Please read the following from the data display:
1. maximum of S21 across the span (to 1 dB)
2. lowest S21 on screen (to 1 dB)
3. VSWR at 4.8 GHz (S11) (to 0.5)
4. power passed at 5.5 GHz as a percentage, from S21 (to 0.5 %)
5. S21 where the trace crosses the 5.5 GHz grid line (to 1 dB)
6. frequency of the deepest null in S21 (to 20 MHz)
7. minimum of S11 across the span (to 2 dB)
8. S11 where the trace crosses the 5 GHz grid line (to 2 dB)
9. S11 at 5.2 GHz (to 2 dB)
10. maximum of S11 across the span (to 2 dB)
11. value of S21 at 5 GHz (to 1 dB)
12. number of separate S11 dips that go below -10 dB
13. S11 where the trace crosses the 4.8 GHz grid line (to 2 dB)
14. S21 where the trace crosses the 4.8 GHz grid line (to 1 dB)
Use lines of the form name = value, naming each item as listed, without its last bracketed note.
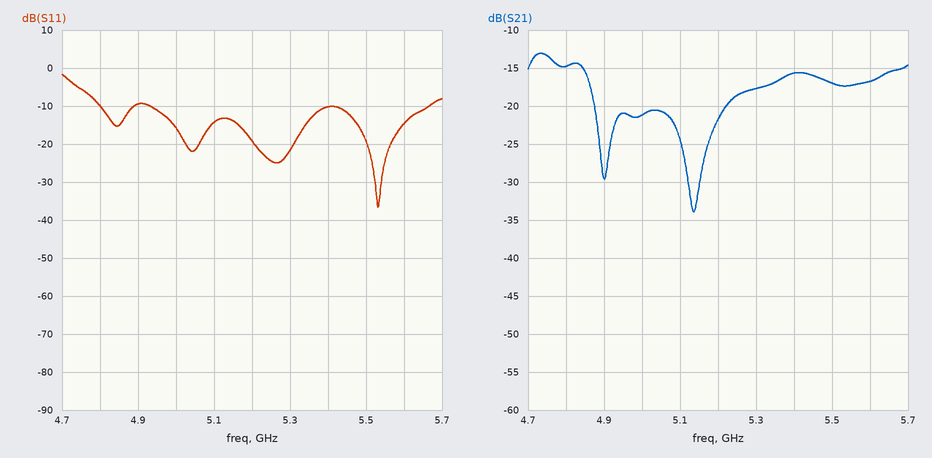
maximum of S21 across the span = -13 dB
lowest S21 on screen = -34 dB
VSWR at 4.8 GHz (S11) = 2.0
power passed at 5.5 GHz as a percentage, from S21 = 2.0 %
S21 where the trace crosses the 5.5 GHz grid line = -17 dB
frequency of the deepest null in S21 = 5.14 GHz
minimum of S11 across the span = -36 dB
S11 where the trace crosses the 5 GHz grid line = -16 dB
S11 at 5.2 GHz = -20 dB
maximum of S11 across the span = -2 dB
value of S21 at 5 GHz = -21 dB
number of separate S11 dips that go below -10 dB = 4
S11 where the trace crosses the 4.8 GHz grid line = -10 dB
S21 where the trace crosses the 4.8 GHz grid line = -15 dB
